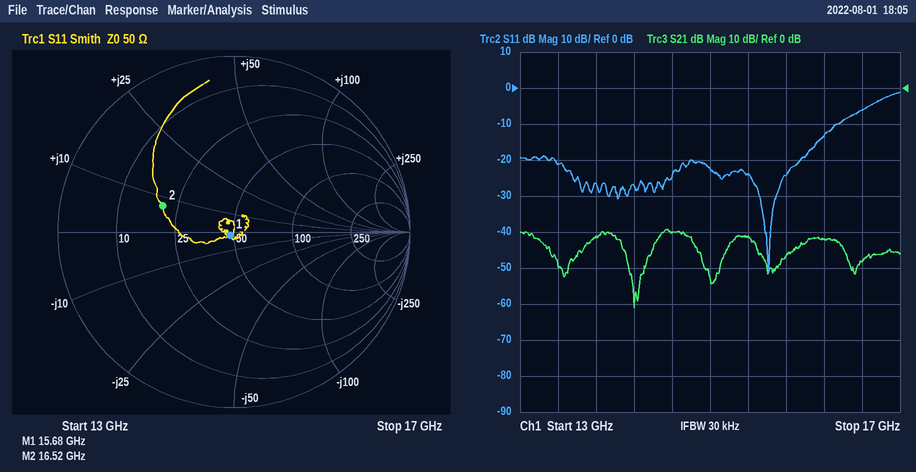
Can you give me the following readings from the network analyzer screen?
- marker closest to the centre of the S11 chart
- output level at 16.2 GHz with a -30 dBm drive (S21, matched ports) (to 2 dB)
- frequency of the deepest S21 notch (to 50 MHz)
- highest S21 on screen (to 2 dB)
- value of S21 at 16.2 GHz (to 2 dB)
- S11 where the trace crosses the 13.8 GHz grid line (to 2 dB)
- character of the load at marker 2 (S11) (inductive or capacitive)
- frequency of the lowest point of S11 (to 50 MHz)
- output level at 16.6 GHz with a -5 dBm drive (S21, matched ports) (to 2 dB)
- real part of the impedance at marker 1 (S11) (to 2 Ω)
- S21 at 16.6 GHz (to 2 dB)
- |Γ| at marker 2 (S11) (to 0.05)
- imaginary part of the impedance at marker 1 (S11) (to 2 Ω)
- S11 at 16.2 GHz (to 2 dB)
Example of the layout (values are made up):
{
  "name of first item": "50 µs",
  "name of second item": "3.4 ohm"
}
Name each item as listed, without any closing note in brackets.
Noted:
{
  "marker closest to the centre of the S11 chart": "marker 1",
  "output level at 16.2 GHz with a -30 dBm drive (S21, matched ports)": "-72 dBm",
  "frequency of the deepest S21 notch": "14.20 GHz",
  "highest S21 on screen": "-40 dB",
  "value of S21 at 16.2 GHz": "-42 dB",
  "S11 where the trace crosses the 13.8 GHz grid line": "-26 dB",
  "character of the load at marker 2 (S11)": "inductive",
  "frequency of the lowest point of S11": "15.60 GHz",
  "output level at 16.6 GHz with a -5 dBm drive (S21, matched ports)": "-54 dBm",
  "real part of the impedance at marker 1 (S11)": "48 Ω",
  "S21 at 16.6 GHz": "-48 dB",
  "|Γ| at marker 2 (S11)": "0.45",
  "imaginary part of the impedance at marker 1 (S11)": "-2 Ω",
  "S11 at 16.2 GHz": "-14 dB"
}
